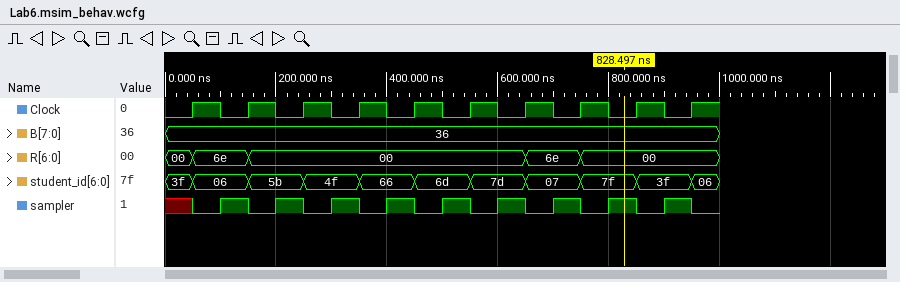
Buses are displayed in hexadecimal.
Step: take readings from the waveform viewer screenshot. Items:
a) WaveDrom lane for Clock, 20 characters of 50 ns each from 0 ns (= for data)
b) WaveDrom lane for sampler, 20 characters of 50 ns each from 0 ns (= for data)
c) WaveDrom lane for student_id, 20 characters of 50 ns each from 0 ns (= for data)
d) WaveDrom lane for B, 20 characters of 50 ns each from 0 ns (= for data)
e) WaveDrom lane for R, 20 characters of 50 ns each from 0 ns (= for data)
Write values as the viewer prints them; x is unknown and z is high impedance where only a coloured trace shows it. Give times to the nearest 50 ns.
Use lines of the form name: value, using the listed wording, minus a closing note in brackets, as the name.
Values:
WaveDrom lane for Clock, 20 characters of 50 ns each from 0 ns: {name: 'Clock', wave: '01010101010101010101'}
WaveDrom lane for sampler, 20 characters of 50 ns each from 0 ns: {name: 'sampler', wave: 'x0101010101010101010'}
WaveDrom lane for student_id, 20 characters of 50 ns each from 0 ns: {name: 'student_id', wave: '==.=.=.=.=.=.=.=.=.=', data: '3f 06 5b 4f 66 6d 7d 07 7f 3f 06'}
WaveDrom lane for B, 20 characters of 50 ns each from 0 ns: {name: 'B', wave: '=...................', data: '36'}
WaveDrom lane for R, 20 characters of 50 ns each from 0 ns: {name: 'R', wave: '==.=.........=.=....', data: '00 6e 00 6e 00'}
